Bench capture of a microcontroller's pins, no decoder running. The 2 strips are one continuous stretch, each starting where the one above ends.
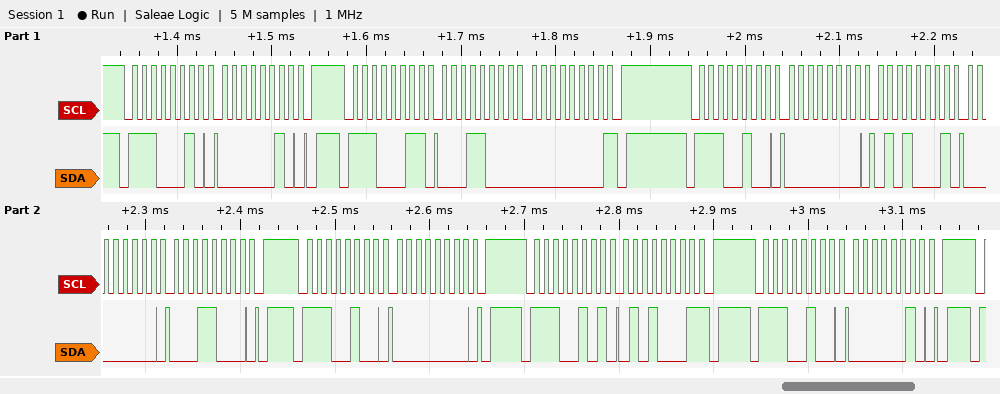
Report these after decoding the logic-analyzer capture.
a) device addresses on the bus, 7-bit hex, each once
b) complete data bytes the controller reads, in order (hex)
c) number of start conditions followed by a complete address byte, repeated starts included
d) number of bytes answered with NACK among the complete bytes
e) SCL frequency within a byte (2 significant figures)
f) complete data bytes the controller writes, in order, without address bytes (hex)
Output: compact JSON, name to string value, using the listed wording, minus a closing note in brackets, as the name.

{"device addresses on the bus, 7-bit hex, each once": "0x71 0x72", "complete data bytes the controller reads, in order": "18 00 51", "number of start conditions followed by a complete address byte, repeated starts included": "6", "number of bytes answered with NACK among the complete bytes": "2", "SCL frequency within a byte": "100 kHz", "complete data bytes the controller writes, in order, without address bytes": "02 00 51 00 18 00 02"}
